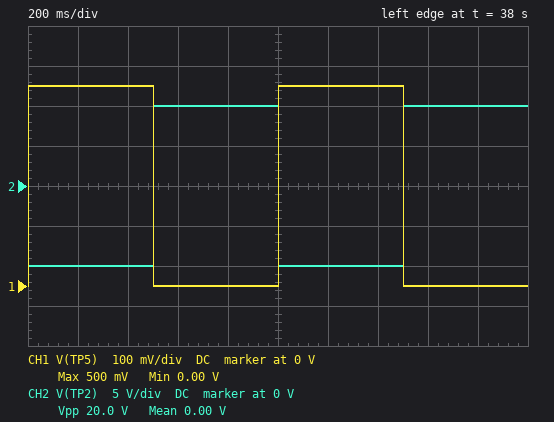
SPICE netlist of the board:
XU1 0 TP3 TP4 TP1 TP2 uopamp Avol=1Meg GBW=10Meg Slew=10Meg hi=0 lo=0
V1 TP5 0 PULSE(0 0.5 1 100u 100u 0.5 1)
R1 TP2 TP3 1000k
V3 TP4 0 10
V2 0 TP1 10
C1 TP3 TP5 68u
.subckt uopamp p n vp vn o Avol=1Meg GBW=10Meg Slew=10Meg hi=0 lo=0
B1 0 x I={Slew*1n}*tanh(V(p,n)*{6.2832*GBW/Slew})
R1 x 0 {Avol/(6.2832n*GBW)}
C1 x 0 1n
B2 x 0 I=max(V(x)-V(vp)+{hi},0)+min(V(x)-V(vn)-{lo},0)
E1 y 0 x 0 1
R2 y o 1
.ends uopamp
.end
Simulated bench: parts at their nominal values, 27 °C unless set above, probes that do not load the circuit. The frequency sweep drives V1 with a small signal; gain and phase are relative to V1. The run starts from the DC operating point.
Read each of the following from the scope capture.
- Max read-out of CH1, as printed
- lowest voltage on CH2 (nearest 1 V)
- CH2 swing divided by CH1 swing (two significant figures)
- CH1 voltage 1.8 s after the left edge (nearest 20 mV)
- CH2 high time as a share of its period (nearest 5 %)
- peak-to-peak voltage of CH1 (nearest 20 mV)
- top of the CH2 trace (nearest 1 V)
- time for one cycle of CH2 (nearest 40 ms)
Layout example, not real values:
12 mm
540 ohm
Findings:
500 mV
-10 V
40
0 V
50 %
500 mV
10 V
1.00 s
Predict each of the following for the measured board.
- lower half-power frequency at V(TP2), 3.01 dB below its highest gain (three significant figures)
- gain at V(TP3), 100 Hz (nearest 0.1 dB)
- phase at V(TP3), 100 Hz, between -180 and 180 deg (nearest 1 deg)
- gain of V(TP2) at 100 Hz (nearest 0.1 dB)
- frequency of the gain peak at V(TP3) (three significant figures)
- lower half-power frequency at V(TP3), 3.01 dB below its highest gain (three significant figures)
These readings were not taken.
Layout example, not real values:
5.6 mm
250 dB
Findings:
148 Hz
-2.5 dB
170 deg
97.4 dB
153 Hz
148 Hz
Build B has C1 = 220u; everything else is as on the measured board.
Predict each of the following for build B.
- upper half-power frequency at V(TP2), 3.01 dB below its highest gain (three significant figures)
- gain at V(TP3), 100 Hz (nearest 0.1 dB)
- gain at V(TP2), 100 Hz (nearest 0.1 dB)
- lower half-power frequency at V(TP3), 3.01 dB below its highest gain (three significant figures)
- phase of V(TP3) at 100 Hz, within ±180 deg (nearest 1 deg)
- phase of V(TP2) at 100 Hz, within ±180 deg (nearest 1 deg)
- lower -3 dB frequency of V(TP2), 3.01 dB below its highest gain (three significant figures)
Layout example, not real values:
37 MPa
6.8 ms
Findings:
90.2 Hz
10.7 dB
110.6 dB
80.7 Hz
14 deg
110 deg
80.2 Hz
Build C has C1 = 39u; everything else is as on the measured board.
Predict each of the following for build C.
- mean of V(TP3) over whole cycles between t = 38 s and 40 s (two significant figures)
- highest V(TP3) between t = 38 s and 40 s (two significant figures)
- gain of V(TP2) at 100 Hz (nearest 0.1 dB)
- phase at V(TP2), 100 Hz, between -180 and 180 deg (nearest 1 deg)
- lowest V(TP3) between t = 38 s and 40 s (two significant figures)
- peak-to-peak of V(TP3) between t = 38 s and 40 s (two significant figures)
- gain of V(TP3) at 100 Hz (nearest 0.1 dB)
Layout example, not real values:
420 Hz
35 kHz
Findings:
67 mV
380 mV
90.2 dB
-92 deg
-250 mV
630 mV
-9.7 dB
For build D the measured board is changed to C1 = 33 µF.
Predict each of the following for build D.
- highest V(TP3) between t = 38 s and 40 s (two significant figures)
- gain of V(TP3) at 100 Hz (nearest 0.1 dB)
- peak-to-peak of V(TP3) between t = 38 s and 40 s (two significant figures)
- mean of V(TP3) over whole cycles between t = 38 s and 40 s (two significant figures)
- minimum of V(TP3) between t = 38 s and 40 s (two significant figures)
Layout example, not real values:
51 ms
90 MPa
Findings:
380 mV
-11.6 dB
660 mV
52 mV
-280 mV
